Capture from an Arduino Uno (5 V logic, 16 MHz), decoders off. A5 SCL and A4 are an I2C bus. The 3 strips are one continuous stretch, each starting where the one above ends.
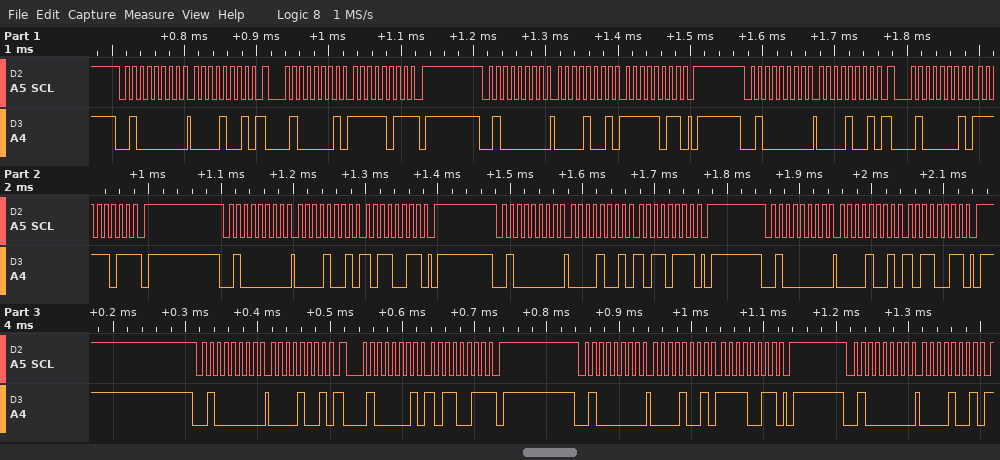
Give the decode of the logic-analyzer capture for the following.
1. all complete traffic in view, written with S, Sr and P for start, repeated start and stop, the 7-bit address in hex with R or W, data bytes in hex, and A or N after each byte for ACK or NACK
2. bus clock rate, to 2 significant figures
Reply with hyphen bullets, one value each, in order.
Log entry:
- S 20W A 09 A Sr 20R A FB N P S 20W A 09 A FB A P S 20W A 09 A Sr 20R A FB N P S 20W A 09 A B3 A P S 20W A 09 A B7 A P S 20W A 09 A B3 A P S 20W A 09 A Sr 20R A B3 N P S 20W A 09 A F3 A P S 20W A 09 A
- 100 kHz
